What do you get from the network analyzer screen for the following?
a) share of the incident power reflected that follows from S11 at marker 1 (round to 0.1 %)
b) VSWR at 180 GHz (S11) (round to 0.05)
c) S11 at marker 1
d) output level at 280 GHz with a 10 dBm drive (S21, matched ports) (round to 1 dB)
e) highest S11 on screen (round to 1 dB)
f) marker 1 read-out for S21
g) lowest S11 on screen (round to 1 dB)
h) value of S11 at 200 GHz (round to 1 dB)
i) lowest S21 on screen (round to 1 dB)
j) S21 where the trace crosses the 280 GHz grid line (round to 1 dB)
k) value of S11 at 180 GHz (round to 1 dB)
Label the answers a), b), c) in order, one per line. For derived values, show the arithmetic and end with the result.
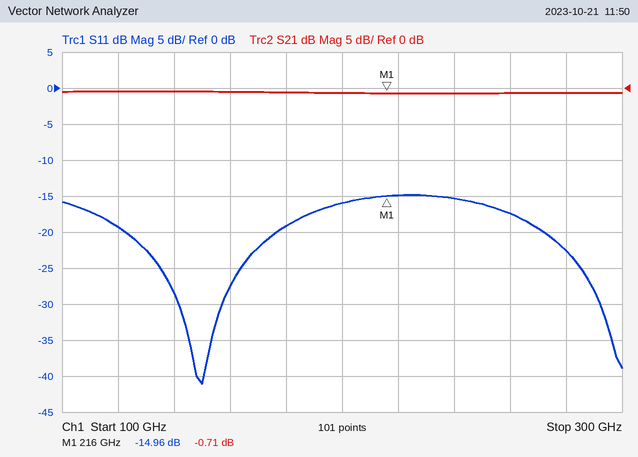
a) 10^(-14.96/10) ≈ 3.2 %
b) |Γ| = 10^(-19/20) = 0.1122; VSWR = (1 + 0.1122)/(1 − 0.1122) ≈ 1.25
c) -14.96 dB
d) 10 dBm + (-1 dB) = 9 dBm
e) -15 dB
f) -0.71 dB
g) -41 dB
h) -16 dB
i) -1 dB
j) -1 dB
k) -19 dB
